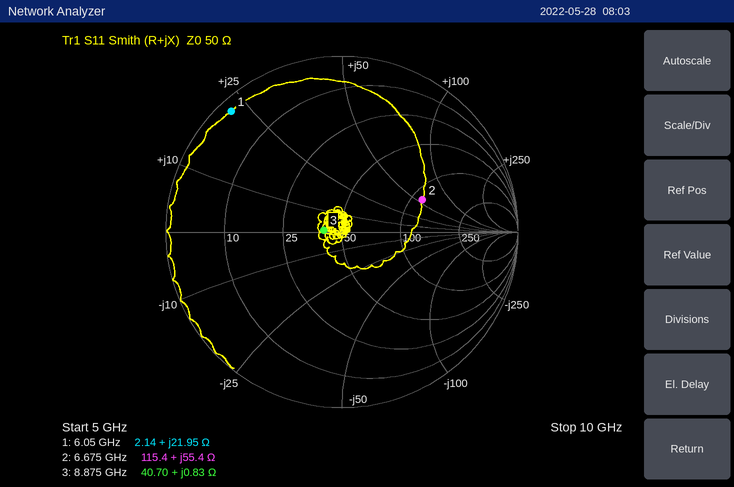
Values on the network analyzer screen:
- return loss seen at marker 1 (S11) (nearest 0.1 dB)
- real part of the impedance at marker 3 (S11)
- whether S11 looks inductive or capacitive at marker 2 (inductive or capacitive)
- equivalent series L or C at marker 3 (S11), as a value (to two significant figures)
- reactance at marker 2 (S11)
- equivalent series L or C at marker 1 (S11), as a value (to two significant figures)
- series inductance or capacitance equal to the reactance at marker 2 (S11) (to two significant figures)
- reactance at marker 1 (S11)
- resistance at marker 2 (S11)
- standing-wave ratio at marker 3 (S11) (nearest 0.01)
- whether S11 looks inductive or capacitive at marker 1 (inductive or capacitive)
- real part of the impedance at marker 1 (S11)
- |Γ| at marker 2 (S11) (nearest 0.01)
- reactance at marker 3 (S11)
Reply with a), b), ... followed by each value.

a) 0.6 dB
b) 40.70 Ω
c) inductive
d) 15 pH
e) +55.4 Ω
f) 580 pH
g) 1.3 nH
h) +21.95 Ω
i) 115.4 Ω
j) 1.23
k) inductive
l) 2.14 Ω
m) 0.49
n) +0.83 Ω
